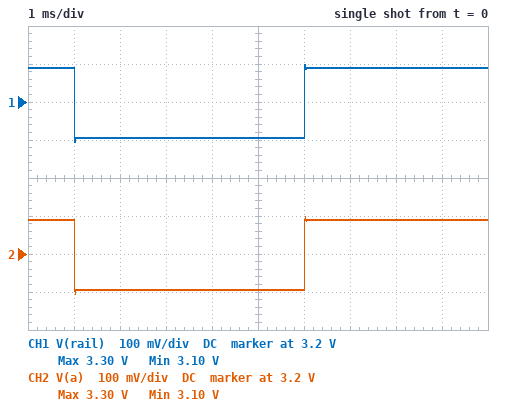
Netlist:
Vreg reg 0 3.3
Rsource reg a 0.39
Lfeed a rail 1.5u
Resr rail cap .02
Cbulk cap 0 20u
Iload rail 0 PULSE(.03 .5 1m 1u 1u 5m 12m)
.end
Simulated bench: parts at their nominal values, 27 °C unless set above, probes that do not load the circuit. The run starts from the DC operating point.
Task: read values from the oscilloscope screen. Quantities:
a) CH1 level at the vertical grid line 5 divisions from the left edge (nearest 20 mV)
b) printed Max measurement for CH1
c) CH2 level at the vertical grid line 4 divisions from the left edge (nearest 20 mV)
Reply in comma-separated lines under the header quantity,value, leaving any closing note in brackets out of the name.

quantity,value
CH1 level at the vertical grid line 5 divisions from the left edge,3.10 V
printed Max measurement for CH1,3.30 V
CH2 level at the vertical grid line 4 divisions from the left edge,3.10 V
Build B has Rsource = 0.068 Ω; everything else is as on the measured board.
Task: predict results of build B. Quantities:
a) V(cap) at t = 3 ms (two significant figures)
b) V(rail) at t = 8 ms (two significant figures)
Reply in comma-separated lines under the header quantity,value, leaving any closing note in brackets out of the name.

quantity,value
V(cap) at t = 3 ms,3.3 V
V(rail) at t = 8 ms,3.3 V
